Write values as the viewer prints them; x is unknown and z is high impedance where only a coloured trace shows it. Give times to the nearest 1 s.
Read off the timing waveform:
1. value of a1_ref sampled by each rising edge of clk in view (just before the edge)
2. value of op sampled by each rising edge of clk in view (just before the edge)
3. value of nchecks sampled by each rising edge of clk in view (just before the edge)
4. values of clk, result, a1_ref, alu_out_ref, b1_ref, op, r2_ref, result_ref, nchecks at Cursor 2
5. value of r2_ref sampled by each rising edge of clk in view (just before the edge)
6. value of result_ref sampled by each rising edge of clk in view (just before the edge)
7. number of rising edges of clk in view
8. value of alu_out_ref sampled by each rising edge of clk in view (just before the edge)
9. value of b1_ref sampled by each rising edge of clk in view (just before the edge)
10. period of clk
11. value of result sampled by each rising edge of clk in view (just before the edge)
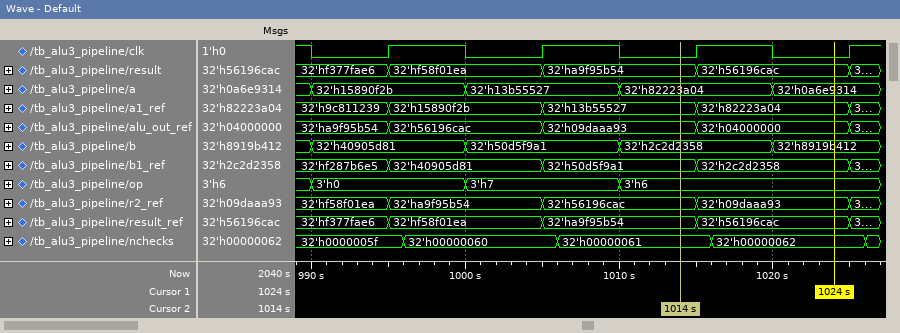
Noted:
32'h9c811239, 32'h15890f2b, 32'h13b55527, 32'h82223a04
3'h0, 3'h7, 3'h6, 3'h6
32'h0000005f, 32'h00000060, 32'h00000061, 32'h00000062
clk=0, result=32'ha9f95b54, a1_ref=32'h13b55527, alu_out_ref=32'h09daaa93, b1_ref=32'h50d5f9a1, op=3'h6, r2_ref=32'h56196cac, result_ref=32'ha9f95b54, nchecks=32'h00000061
32'hf58f01ea, 32'ha9f95b54, 32'h56196cac, 32'h09daaa93
32'hf377fae6, 32'hf58f01ea, 32'ha9f95b54, 32'h56196cac
4
32'ha9f95b54, 32'h56196cac, 32'h09daaa93, 32'h04000000
32'hf287b6e5, 32'h40905d81, 32'h50d5f9a1, 32'h2c2d2358
10 s
32'hf377fae6, 32'hf58f01ea, 32'ha9f95b54, 32'h56196cac
